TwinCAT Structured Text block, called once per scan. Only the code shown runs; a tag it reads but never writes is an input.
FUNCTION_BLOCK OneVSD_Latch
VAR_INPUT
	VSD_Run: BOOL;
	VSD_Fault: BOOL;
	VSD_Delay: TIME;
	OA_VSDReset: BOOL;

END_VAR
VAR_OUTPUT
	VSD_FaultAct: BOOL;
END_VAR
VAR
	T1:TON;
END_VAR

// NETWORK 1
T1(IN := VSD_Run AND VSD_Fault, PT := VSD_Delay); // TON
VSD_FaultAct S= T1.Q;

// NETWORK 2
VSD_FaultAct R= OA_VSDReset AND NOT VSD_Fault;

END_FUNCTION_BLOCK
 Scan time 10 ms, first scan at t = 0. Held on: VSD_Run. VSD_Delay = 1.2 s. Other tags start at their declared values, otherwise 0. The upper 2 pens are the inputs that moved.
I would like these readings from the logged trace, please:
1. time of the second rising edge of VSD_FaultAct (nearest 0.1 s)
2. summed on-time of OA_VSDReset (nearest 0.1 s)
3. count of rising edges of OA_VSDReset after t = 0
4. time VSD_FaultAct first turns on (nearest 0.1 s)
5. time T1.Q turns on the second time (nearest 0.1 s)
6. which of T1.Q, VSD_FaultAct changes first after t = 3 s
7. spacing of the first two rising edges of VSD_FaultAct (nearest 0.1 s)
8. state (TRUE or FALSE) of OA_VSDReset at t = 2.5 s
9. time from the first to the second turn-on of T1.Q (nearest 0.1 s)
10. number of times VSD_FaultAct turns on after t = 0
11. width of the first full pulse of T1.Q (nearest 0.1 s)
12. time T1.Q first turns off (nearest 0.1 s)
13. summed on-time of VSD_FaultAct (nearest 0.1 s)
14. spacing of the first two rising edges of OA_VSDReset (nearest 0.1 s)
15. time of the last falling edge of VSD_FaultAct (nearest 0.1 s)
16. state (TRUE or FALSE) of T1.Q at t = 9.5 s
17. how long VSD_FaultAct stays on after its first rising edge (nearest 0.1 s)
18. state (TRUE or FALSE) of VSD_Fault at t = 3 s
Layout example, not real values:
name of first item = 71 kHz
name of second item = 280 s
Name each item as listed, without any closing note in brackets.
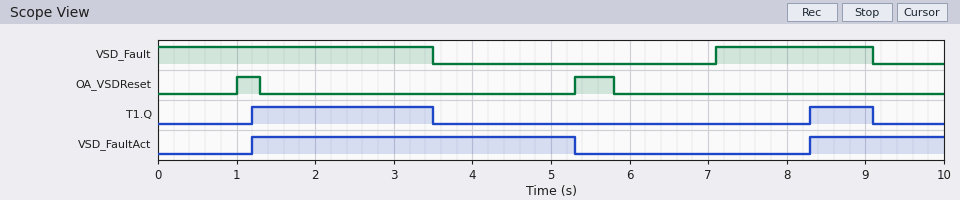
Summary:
time of the second rising edge of VSD_FaultAct = 8.3 s
summed on-time of OA_VSDReset = 0.8 s
count of rising edges of OA_VSDReset after t = 0 = 2
time VSD_FaultAct first turns on = 1.2 s
time T1.Q turns on the second time = 8.3 s
which of T1.Q, VSD_FaultAct changes first after t = 3 s = T1.Q
spacing of the first two rising edges of VSD_FaultAct = 7.1 s
state (TRUE or FALSE) of OA_VSDReset at t = 2.5 s = FALSE
time from the first to the second turn-on of T1.Q = 7.1 s
number of times VSD_FaultAct turns on after t = 0 = 2
width of the first full pulse of T1.Q = 2.3 s
time T1.Q first turns off = 3.5 s
summed on-time of VSD_FaultAct = 5.8 s
spacing of the first two rising edges of OA_VSDReset = 4.3 s
time of the last falling edge of VSD_FaultAct = 5.3 s
state (TRUE or FALSE) of T1.Q at t = 9.5 s = FALSE
how long VSD_FaultAct stays on after its first rising edge = 4.1 s
state (TRUE or FALSE) of VSD_Fault at t = 3 s = TRUE
